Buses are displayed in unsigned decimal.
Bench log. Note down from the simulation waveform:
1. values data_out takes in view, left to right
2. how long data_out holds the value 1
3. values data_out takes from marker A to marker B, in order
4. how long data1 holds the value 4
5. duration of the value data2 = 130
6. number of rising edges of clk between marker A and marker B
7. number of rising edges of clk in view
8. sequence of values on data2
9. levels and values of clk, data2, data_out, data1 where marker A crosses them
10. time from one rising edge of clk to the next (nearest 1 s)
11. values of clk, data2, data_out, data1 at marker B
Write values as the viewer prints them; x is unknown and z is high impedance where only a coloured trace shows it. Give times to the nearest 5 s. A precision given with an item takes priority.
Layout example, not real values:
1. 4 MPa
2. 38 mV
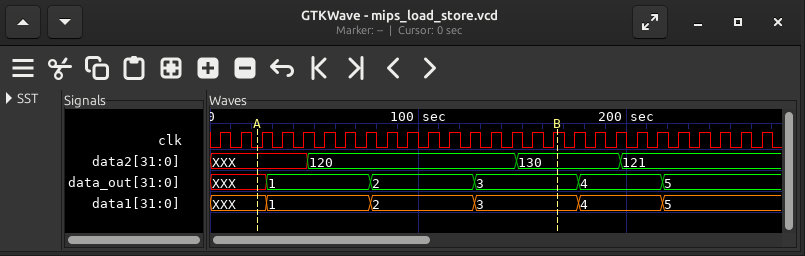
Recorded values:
1. XXX, 1, 2, 3, 4, 5
2. 50 s
3. XXX, 1, 2, 3
4. 40 s
5. 50 s
6. 15
7. 27
8. XXX, 120, 130, 121
9. clk=0, data2=XXX, data_out=XXX, data1=XXX
10. 10 s
11. clk=1, data2=130, data_out=3, data1=3
